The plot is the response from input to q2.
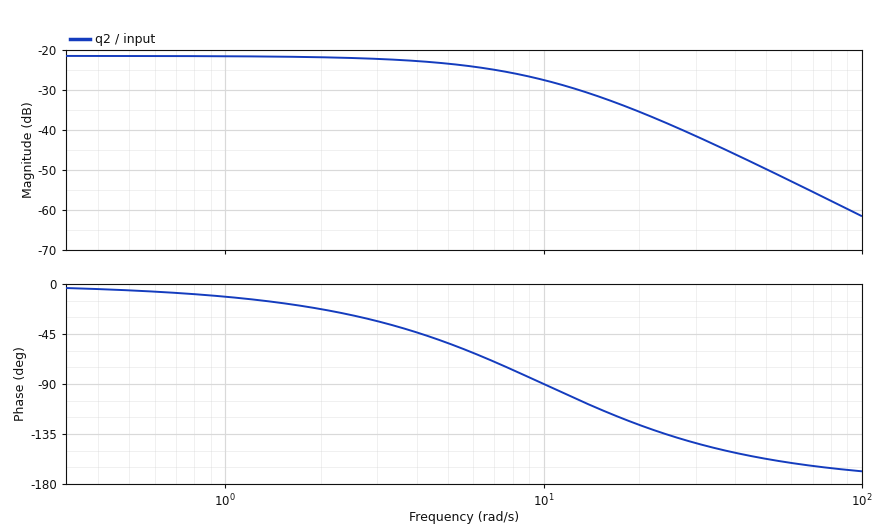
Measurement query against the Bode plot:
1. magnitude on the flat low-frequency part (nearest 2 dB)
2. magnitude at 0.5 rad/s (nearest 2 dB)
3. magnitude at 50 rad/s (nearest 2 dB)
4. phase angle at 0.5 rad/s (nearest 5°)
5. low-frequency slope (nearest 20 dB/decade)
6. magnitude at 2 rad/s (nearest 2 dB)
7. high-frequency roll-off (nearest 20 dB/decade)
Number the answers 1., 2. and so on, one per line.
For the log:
1. -22 dB
2. -22 dB
3. -50 dB
4. -5°
5. 0 dB/decade
6. -22 dB
7. -40 dB/decade
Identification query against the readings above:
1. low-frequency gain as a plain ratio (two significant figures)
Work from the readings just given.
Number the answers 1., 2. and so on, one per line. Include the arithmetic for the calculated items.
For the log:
1. 10^(-22 / 20) = 0.079
